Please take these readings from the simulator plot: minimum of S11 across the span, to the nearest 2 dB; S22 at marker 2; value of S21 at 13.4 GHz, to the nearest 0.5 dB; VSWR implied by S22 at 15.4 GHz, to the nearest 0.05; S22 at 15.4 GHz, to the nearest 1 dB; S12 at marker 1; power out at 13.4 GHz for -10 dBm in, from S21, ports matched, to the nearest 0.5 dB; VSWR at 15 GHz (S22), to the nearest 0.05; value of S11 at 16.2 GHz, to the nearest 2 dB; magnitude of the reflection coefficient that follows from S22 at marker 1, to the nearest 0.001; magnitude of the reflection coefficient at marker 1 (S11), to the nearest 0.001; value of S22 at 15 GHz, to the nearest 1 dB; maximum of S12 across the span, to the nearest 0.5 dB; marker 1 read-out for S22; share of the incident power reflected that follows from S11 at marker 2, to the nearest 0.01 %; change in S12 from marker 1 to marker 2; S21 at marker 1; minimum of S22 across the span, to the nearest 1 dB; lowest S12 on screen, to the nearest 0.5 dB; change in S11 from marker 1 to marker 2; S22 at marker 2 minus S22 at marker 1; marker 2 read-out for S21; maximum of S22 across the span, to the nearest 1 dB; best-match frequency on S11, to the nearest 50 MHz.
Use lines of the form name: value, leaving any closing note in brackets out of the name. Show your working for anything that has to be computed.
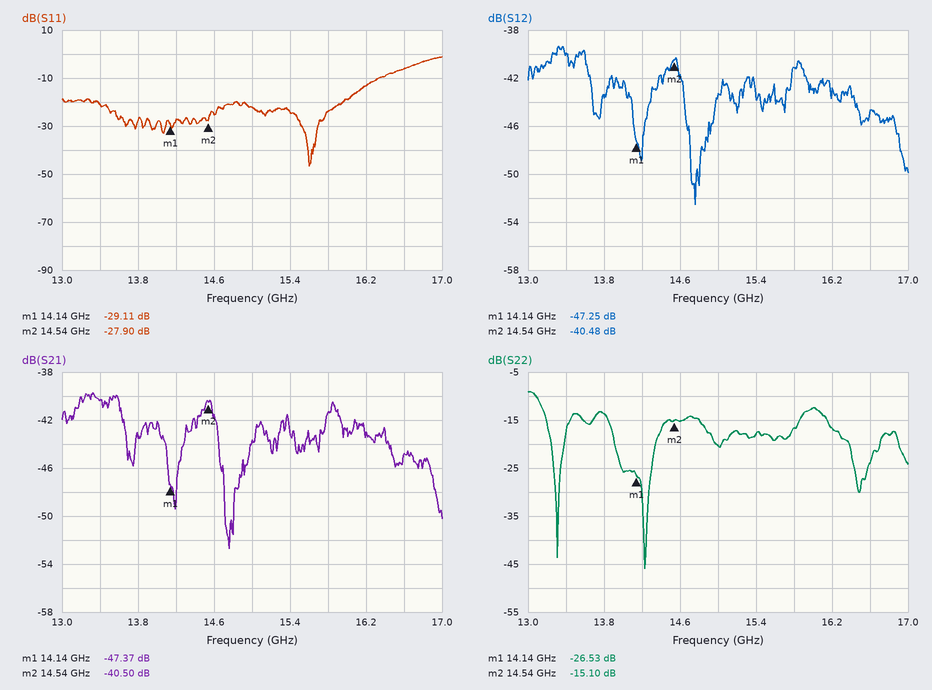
minimum of S11 across the span, to the nearest 2 dB: -46 dB
S22 at marker 2: -15.10 dB
value of S21 at 13.4 GHz, to the nearest 0.5 dB: -40.5 dB
VSWR implied by S22 at 15.4 GHz, to the nearest 0.05: |Γ| = 10^(-18/20) = 0.1259; VSWR = (1 + 0.1259)/(1 − 0.1259) ≈ 1.29, so 1.30 to the nearest 0.05
S22 at 15.4 GHz, to the nearest 1 dB: -18 dB
S12 at marker 1: -47.25 dB
power out at 13.4 GHz for -10 dBm in, from S21, ports matched, to the nearest 0.5 dB: -10 dBm + (-40.5 dB) = -50.5 dBm
VSWR at 15 GHz (S22), to the nearest 0.05: |Γ| = 10^(-20/20) = 0.1000; VSWR = (1 + 0.1000)/(1 − 0.1000) ≈ 1.22, so 1.20 to the nearest 0.05
value of S11 at 16.2 GHz, to the nearest 2 dB: -14 dB
magnitude of the reflection coefficient that follows from S22 at marker 1, to the nearest 0.001: 10^(-26.53/20) ≈ 0.047
magnitude of the reflection coefficient at marker 1 (S11), to the nearest 0.001: 10^(-29.11/20) ≈ 0.035
value of S22 at 15 GHz, to the nearest 1 dB: -20 dB
maximum of S12 across the span, to the nearest 0.5 dB: -39.5 dB
marker 1 read-out for S22: -26.53 dB
share of the incident power reflected that follows from S11 at marker 2, to the nearest 0.01 %: 10^(-27.9/10) ≈ 0.16 %
change in S12 from marker 1 to marker 2: -40.48 − (-47.25) = 6.77 dB
S21 at marker 1: -47.37 dB
minimum of S22 across the span, to the nearest 1 dB: -46 dB
lowest S12 on screen, to the nearest 0.5 dB: -52.5 dB
change in S11 from marker 1 to marker 2: -27.9 − (-29.11) = 1.21 dB
S22 at marker 2 minus S22 at marker 1: -15.1 − (-26.53) = 11.43 dB
marker 2 read-out for S21: -40.50 dB
maximum of S22 across the span, to the nearest 1 dB: -9 dB
best-match frequency on S11, to the nearest 50 MHz: 15.60 GHz
